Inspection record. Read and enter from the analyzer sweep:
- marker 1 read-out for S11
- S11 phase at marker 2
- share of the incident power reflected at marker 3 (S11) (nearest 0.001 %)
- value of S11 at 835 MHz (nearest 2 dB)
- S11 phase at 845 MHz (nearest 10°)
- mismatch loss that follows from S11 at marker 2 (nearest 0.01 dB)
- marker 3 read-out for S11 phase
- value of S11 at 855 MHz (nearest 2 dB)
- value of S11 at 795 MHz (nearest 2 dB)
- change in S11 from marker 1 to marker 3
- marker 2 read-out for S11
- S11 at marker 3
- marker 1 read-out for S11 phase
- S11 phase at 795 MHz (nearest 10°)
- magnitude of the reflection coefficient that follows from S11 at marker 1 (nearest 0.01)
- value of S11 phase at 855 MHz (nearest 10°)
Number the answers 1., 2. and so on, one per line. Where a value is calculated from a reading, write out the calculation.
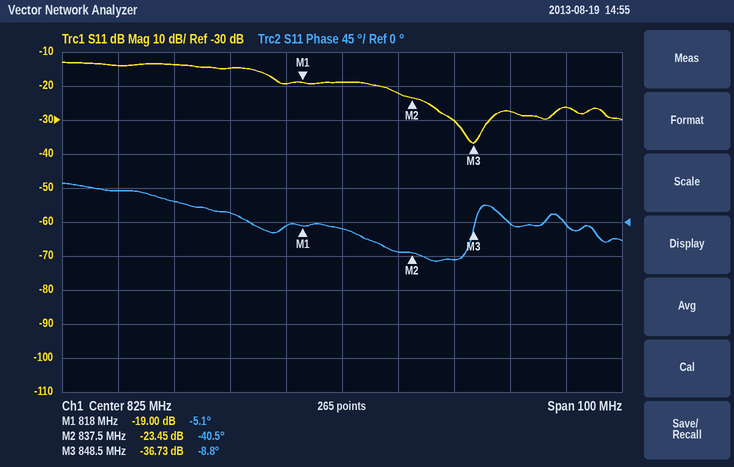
1. -19.00 dB
2. -40.5°
3. 10^(-36.73/10) ≈ 0.021 %
4. -22 dB
5. -50°
6. −10 log10(1 − 10^(-23.45/10)) ≈ 0.02 dB
7. -8.8°
8. -28 dB
9. -14 dB
10. -36.73 − (-19) = -17.73 dB
11. -23.45 dB
12. -36.73 dB
13. -5.1°
14. 30°
15. 10^(-19/20) ≈ 0.11
16. 0°
